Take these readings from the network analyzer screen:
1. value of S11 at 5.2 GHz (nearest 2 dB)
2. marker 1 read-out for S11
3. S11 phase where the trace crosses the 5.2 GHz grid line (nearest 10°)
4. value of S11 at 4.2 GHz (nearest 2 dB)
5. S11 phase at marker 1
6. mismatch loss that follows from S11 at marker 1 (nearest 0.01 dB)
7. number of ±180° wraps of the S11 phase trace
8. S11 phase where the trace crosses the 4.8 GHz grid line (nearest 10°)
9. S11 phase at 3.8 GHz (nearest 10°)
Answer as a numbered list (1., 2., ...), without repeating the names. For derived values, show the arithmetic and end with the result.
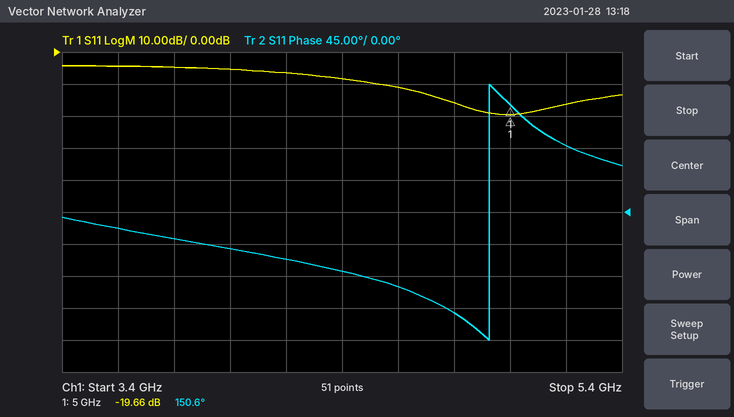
1. -16 dB
2. -19.66 dB
3. 90°
4. -6 dB
5. 150.6°
6. −10 log10(1 − 10^(-19.66/10)) ≈ 0.05 dB
7. 1
8. -140°
9. -40°
